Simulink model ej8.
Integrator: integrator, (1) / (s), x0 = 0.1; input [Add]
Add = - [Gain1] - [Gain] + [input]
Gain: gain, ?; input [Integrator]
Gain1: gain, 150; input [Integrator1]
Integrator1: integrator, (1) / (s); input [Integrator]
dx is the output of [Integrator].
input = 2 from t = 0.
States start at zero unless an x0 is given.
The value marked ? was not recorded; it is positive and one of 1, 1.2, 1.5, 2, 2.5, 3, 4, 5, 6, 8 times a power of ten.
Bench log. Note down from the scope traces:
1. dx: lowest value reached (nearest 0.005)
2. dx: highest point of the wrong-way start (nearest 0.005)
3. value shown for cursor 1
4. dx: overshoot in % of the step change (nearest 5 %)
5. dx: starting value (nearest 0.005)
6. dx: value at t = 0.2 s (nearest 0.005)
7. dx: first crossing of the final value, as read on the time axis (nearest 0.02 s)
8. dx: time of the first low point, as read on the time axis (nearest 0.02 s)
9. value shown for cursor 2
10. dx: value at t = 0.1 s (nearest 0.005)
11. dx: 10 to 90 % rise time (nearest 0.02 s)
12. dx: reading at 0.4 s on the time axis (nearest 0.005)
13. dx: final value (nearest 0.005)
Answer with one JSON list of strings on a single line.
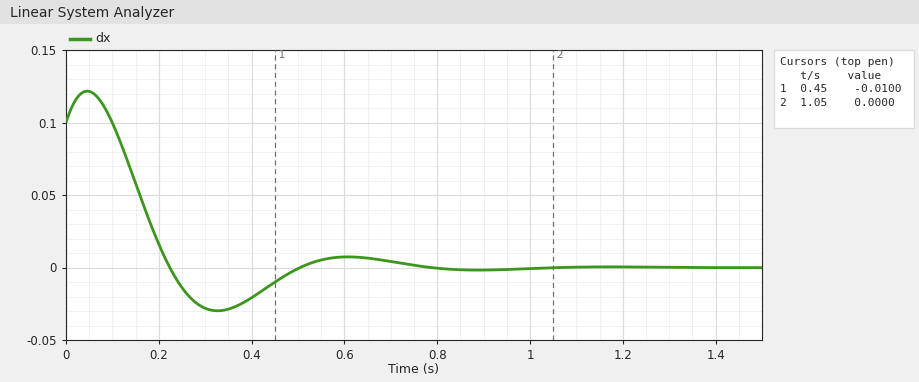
["-0.030", "0.120", "-0.0100", "30 %", "0.100", "0.015", "0.22 s", "0.32 s", "0.0000", "0.100", "0.10 s", "-0.020", "0.000"]
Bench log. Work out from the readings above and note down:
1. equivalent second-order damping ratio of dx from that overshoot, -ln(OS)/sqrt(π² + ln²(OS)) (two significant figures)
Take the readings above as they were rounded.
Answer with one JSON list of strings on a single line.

["0.36"]
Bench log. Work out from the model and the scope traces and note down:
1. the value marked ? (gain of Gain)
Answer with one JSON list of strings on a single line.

["10"]
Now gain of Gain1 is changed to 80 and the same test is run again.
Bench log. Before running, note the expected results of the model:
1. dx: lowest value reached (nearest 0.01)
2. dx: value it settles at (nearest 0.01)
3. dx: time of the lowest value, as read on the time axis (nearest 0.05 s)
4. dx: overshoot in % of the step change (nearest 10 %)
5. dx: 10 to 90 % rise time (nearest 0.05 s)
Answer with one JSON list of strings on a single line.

["-0.02", "0.00", "0.50 s", "20 %", "0.15 s"]
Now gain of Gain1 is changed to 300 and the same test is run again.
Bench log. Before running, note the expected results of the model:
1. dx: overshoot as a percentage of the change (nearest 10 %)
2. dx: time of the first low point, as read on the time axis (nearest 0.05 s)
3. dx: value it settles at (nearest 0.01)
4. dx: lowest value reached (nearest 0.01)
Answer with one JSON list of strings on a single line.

["40 %", "0.20 s", "0.00", "-0.04"]
